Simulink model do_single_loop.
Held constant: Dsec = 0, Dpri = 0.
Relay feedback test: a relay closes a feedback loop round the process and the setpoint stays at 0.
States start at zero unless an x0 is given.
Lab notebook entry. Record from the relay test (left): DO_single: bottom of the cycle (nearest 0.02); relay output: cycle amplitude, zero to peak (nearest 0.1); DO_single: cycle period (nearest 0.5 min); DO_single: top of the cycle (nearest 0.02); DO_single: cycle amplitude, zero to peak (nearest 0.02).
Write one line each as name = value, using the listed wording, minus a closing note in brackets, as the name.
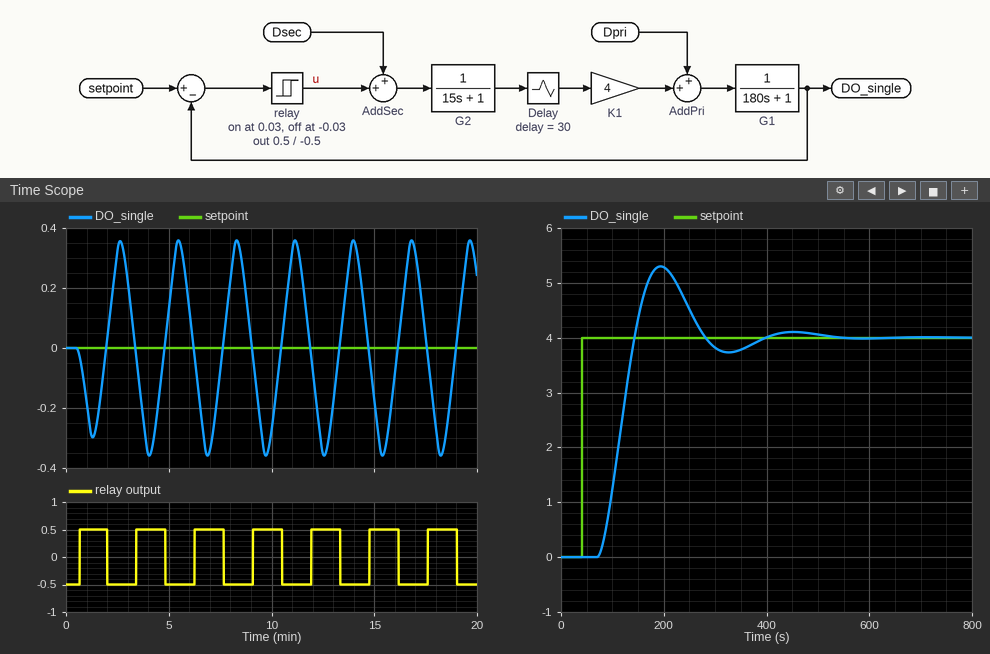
DO_single: bottom of the cycle = -0.36
relay output: cycle amplitude, zero to peak = 0.5
DO_single: cycle period = 3.0 min
DO_single: top of the cycle = 0.36
DO_single: cycle amplitude, zero to peak = 0.36
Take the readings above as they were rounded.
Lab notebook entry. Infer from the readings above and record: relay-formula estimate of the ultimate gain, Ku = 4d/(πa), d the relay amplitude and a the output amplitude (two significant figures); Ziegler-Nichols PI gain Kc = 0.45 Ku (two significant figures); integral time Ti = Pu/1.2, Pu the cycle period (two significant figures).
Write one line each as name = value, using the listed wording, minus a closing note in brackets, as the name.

relay-formula estimate of the ultimate gain, Ku = 4d/(πa), d the relay amplitude and a the output amplitude = 1.8
Ziegler-Nichols PI gain Kc = 0.45 Ku = 0.81
integral time Ti = Pu/1.2, Pu the cycle period = 2.5 min
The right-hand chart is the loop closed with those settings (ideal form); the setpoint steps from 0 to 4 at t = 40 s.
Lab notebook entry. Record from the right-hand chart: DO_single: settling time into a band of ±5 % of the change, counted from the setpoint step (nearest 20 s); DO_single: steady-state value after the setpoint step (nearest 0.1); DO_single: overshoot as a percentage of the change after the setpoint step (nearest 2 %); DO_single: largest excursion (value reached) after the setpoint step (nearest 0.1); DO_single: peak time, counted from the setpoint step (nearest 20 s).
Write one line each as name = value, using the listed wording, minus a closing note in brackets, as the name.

DO_single: settling time into a band of ±5 % of the change, counted from the setpoint step = 320 s
DO_single: steady-state value after the setpoint step = 4.0
DO_single: overshoot as a percentage of the change after the setpoint step = 32 %
DO_single: largest excursion (value reached) after the setpoint step = 5.3
DO_single: peak time, counted from the setpoint step = 160 s
